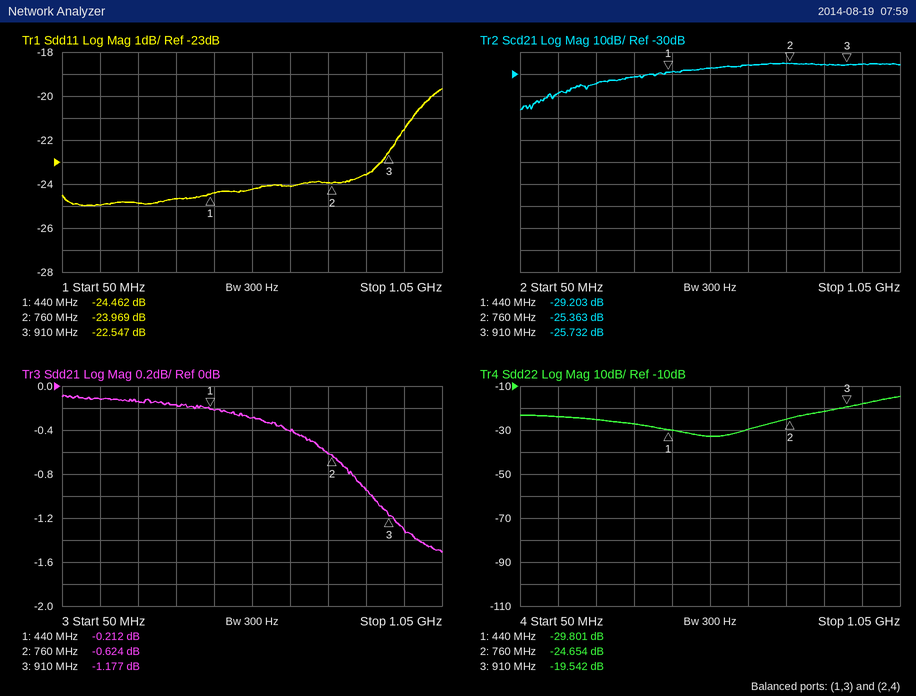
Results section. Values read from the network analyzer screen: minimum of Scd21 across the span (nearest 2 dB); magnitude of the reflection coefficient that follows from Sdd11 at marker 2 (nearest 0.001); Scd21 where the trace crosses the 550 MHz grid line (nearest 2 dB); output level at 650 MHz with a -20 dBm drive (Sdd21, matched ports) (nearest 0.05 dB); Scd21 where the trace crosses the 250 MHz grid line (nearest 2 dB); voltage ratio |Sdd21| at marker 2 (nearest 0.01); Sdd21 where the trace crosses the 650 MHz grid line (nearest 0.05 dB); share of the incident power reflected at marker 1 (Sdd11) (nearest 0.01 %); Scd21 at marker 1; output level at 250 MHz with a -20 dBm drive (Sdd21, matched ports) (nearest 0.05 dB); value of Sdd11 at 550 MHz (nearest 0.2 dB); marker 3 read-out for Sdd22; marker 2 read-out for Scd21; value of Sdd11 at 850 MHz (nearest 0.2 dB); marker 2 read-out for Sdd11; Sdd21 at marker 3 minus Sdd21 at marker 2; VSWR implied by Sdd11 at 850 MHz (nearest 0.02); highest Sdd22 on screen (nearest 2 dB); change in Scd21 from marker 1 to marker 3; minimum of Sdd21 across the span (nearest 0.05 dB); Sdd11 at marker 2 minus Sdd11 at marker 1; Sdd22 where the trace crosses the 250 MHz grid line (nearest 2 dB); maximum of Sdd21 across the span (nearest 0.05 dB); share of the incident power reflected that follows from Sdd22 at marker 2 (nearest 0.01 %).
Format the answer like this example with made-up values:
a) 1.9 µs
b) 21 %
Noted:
a) -46 dB
b) 0.063
c) -28 dB
d) -20.40 dBm
e) -34 dB
f) 0.93
g) -0.40 dB
h) 0.36 %
i) -29.203 dB
j) -20.15 dBm
k) -24.2 dB
l) -19.542 dB
m) -25.363 dB
n) -23.6 dB
o) -23.969 dB
p) -0.553 dB
q) 1.14
r) -14 dB
s) 3.471 dB
t) -1.50 dB
u) 0.493 dB
v) -26 dB
w) -0.10 dB
x) 0.34 %
